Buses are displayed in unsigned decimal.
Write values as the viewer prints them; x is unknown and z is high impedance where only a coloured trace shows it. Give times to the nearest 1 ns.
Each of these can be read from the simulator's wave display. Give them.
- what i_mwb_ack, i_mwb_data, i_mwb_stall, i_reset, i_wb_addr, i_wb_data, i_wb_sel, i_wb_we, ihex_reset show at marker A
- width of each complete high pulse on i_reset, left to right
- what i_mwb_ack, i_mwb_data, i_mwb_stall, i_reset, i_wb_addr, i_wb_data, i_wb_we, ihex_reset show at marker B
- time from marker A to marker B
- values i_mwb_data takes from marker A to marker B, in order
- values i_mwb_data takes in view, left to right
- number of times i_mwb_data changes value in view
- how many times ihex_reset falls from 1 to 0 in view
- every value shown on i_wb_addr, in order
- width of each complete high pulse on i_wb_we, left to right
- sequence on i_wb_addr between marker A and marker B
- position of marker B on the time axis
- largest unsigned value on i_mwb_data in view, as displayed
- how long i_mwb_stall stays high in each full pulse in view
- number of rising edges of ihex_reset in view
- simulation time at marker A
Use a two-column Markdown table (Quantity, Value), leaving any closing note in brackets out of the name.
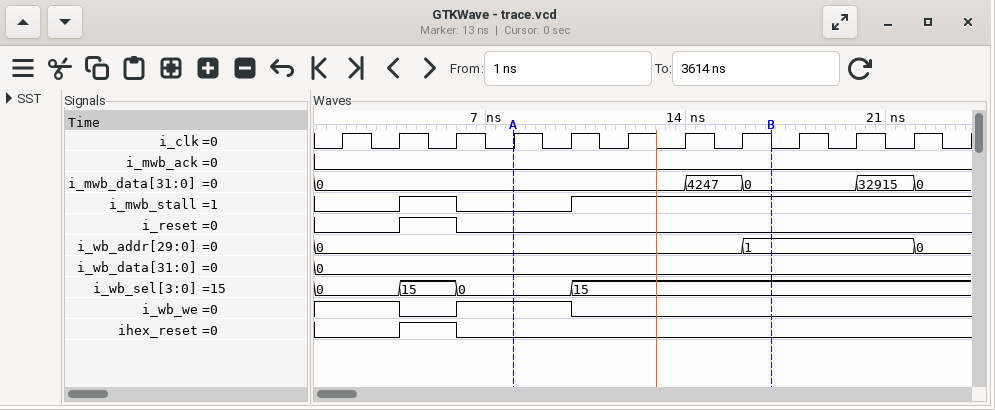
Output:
| Quantity | Value |
|---|---|
| what i_mwb_ack, i_mwb_data, i_mwb_stall, i_reset, i_wb_addr, i_wb_data, i_wb_sel, i_wb_we, ihex_reset show at marker A | i_mwb_ack=0, i_mwb_data=0, i_mwb_stall=0, i_reset=0, i_wb_addr=0, i_wb_data=0, i_wb_sel=0, i_wb_we=1, ihex_reset=0 |
| width of each complete high pulse on i_reset, left to right | 2 ns |
| what i_mwb_ack, i_mwb_data, i_mwb_stall, i_reset, i_wb_addr, i_wb_data, i_wb_we, ihex_reset show at marker B | i_mwb_ack=0, i_mwb_data=0, i_mwb_stall=1, i_reset=0, i_wb_addr=1, i_wb_data=0, i_wb_we=0, ihex_reset=0 |
| time from marker A to marker B | 9 ns |
| values i_mwb_data takes from marker A to marker B, in order | 0, 4247, 0 |
| values i_mwb_data takes in view, left to right | 0, 4247, 0, 32915, 0 |
| number of times i_mwb_data changes value in view | 4 |
| how many times ihex_reset falls from 1 to 0 in view | 1 |
| every value shown on i_wb_addr, in order | 0, 1, 0 |
| width of each complete high pulse on i_wb_we, left to right | 4 ns |
| sequence on i_wb_addr between marker A and marker B | 0, 1 |
| position of marker B on the time axis | 17 ns |
| largest unsigned value on i_mwb_data in view, as displayed | 32915 |
| how long i_mwb_stall stays high in each full pulse in view | 2 ns |
| number of rising edges of ihex_reset in view | 1 |
| simulation time at marker A | 8 ns |
